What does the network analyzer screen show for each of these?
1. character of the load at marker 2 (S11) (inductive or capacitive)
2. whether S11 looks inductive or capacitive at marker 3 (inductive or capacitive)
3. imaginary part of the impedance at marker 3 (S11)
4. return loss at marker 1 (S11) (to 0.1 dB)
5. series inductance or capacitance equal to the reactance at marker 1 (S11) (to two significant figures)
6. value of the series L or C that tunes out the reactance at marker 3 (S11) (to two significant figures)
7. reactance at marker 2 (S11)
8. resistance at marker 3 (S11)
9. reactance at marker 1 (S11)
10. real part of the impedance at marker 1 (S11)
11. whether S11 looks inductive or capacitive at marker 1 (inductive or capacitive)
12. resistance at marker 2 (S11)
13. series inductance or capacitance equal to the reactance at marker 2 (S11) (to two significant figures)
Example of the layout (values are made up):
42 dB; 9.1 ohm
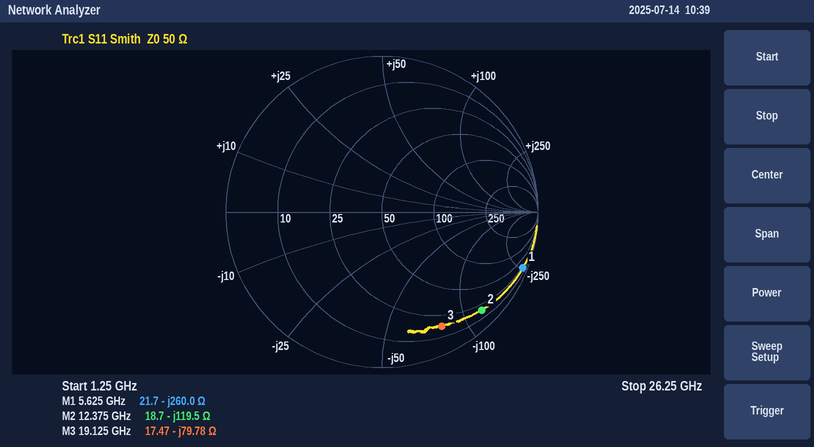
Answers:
capacitive; capacitive; -79.78 Ω; 0.3 dB; 110 fF; 660 pH; -119.5 Ω; 17.47 Ω; -260.0 Ω; 21.7 Ω; capacitive; 18.7 Ω; 110 fF
